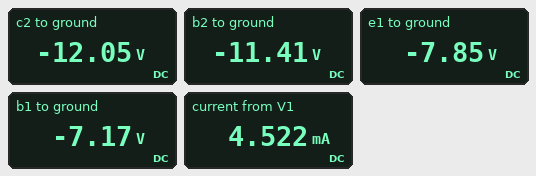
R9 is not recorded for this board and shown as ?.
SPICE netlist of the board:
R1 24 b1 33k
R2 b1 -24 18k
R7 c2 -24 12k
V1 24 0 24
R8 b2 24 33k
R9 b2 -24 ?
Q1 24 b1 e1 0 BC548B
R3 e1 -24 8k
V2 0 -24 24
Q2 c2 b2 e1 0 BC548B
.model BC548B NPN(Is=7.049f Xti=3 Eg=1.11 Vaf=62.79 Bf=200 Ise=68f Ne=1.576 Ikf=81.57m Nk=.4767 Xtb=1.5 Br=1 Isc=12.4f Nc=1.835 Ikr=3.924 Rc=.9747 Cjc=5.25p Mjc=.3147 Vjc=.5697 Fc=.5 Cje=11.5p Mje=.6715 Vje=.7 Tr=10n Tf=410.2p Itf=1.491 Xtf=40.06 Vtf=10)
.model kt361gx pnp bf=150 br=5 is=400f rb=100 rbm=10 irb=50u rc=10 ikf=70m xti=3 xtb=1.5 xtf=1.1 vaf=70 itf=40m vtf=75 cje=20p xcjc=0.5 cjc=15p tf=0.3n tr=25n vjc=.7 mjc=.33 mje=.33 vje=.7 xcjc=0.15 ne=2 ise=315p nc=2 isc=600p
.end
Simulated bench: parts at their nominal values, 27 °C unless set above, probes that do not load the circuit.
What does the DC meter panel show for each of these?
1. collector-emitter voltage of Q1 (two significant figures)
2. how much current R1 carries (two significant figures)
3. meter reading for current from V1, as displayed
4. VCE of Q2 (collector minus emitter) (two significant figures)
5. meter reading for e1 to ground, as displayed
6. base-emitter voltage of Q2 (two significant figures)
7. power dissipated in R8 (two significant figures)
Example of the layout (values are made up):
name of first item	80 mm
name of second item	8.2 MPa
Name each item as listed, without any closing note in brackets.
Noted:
collector-emitter voltage of Q1	32 V
how much current R1 carries	940 µA
meter reading for current from V1, as displayed	4.522 mA
VCE of Q2 (collector minus emitter)	-4.2 V
meter reading for e1 to ground, as displayed	-7.85 V
base-emitter voltage of Q2	-3.6 V
power dissipated in R8	38 mW
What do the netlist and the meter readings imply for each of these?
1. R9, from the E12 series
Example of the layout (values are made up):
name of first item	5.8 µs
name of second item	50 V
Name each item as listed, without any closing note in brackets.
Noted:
R9, from the E12 series	22 kΩ
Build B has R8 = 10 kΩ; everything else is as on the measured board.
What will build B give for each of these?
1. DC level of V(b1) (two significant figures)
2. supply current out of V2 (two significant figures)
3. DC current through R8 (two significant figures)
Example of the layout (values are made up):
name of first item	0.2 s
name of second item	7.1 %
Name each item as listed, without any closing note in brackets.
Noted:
DC level of V(b1)	-7.1 V
supply current out of V2	5.1 mA
DC current through R8	3.1 mA
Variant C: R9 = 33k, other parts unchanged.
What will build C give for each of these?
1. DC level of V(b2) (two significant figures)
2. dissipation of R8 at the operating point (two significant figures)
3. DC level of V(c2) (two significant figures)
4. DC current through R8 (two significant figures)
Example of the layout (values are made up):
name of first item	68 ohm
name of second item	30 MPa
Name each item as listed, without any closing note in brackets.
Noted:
DC level of V(b2)	-9.5 V
dissipation of R8 at the operating point	34 mW
DC level of V(c2)	-10 V
DC current through R8	1.0 mA
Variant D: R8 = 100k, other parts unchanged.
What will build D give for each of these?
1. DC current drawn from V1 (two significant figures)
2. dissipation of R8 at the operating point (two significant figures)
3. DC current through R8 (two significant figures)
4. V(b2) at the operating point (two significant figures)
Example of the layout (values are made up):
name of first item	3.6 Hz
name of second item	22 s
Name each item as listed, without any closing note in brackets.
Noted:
DC current drawn from V1	3.6 mA
dissipation of R8 at the operating point	18 mW
DC current through R8	430 µA
V(b2) at the operating point	-19 V
